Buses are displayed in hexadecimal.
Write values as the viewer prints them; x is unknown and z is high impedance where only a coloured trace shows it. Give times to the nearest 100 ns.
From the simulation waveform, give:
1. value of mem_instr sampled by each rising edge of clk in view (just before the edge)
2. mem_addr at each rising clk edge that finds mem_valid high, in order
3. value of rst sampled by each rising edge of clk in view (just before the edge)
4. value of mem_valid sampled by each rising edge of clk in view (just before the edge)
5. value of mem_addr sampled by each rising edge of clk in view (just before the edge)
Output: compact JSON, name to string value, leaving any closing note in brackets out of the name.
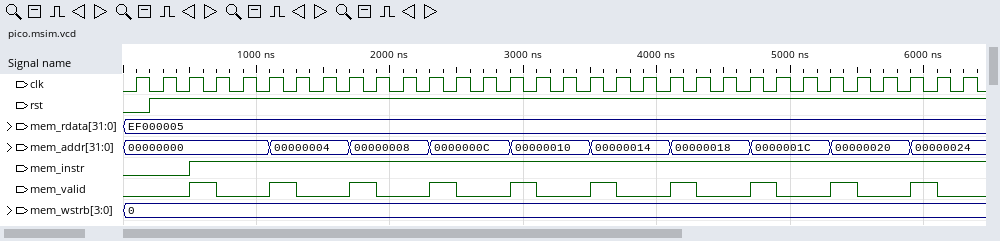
{"value of mem_instr sampled by each rising edge of clk in view": "0 0 0 1 1 1 1 1 1 1 1 1 1 1 1 1 1 1 1 1 1 1 1 1 1 1 1 1 1 1 1 1", "mem_addr at each rising clk edge that finds mem_valid high, in order": "00000000, 00000004, 00000008, 0000000C, 00000010, 00000014, 00000018, 0000001C, 00000020, 00000024", "value of rst sampled by each rising edge of clk in view": "0 1 1 1 1 1 1 1 1 1 1 1 1 1 1 1 1 1 1 1 1 1 1 1 1 1 1 1 1 1 1 1", "value of mem_valid sampled by each rising edge of clk in view": "0 0 0 1 0 0 1 0 0 1 0 0 1 0 0 1 0 0 1 0 0 1 0 0 1 0 0 1 0 0 1 0", "value of mem_addr sampled by each rising edge of clk in view": "00000000, 00000000, 00000000, 00000000, 00000000, 00000000, 00000004, 00000004, 00000004, 00000008, 00000008, 00000008, 0000000C, 0000000C, 0000000C, 00000010, 00000010, 00000010, 00000014, 00000014, 00000014, 00000018, 00000018, 00000018, 0000001C, 0000001C, 0000001C, 00000020, 00000020, 00000020, 00000024, 00000024"}
